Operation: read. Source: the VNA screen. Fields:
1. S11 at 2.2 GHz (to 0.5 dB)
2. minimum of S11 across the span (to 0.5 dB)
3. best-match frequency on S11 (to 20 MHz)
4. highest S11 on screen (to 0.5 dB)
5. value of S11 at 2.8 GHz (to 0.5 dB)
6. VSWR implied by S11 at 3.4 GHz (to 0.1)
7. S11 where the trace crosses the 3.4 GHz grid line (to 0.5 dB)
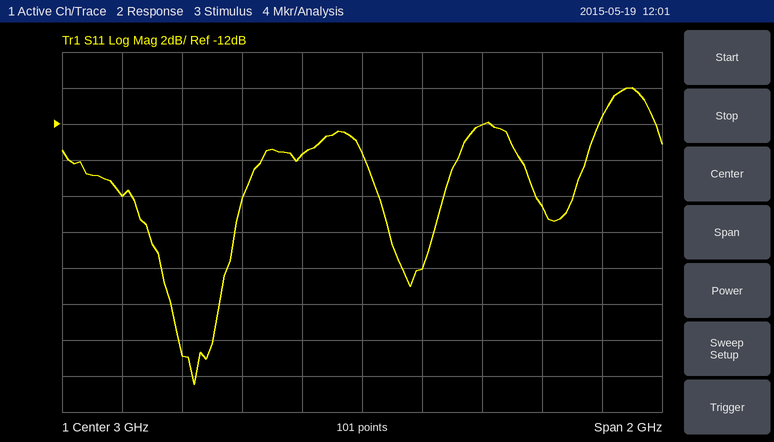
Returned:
-16.0 dB
-26.5 dB
2.44 GHz
-10.0 dB
-13.5 dB
1.7
-12.0 dB
